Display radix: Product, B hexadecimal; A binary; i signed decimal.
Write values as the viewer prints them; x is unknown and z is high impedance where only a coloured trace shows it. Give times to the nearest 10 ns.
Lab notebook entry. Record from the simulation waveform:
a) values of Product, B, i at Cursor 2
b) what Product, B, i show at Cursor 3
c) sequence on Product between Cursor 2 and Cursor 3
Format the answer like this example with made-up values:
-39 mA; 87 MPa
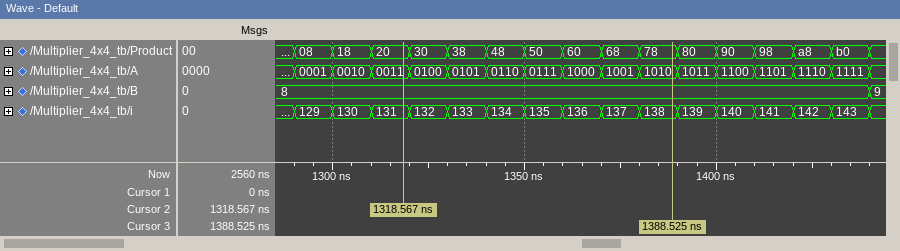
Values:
Product=20, B=8, i=131; Product=78, B=8, i=138; 20, 30, 38, 48, 50, 60, 68, 78
